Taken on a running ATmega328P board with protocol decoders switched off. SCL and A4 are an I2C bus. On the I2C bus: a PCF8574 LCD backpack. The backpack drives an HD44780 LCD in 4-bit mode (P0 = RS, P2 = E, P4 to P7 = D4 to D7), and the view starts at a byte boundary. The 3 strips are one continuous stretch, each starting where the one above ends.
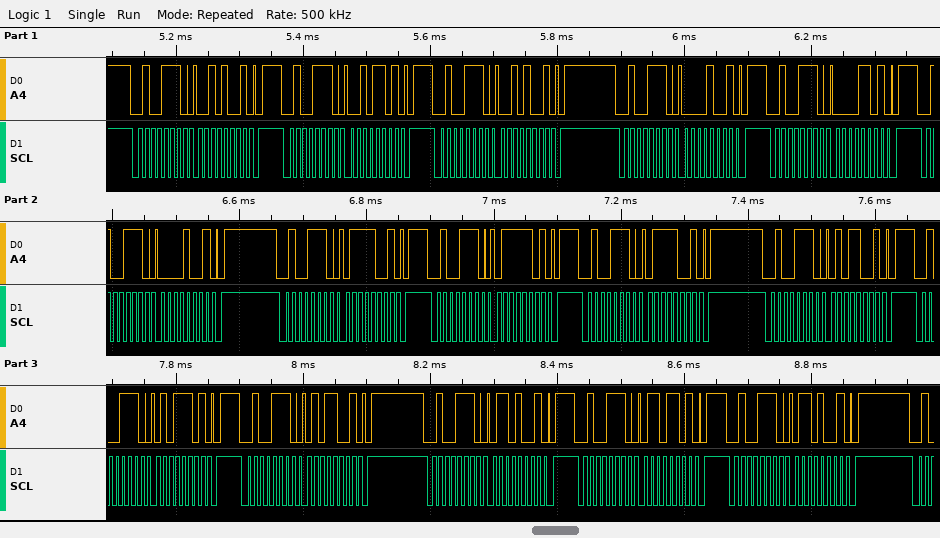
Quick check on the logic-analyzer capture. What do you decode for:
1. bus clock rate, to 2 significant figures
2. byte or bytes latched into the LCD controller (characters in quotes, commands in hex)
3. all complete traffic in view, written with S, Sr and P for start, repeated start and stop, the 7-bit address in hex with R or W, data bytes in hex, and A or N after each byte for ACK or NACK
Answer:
100 kHz
' ' 'u'
S 27W A 29 A P S 27W A 2D A P S 27W A 29 A P S 27W A 09 A P S 27W A 0D A P S 27W A 09 A P S 27W A 79 A P S 27W A 7D A P S 27W A 79 A P S 27W A 59 A P S 27W A 5D A P S 27W A 59 A P S 27W A 69 A P S 27W A 6D A P S 27W A 69 A P
